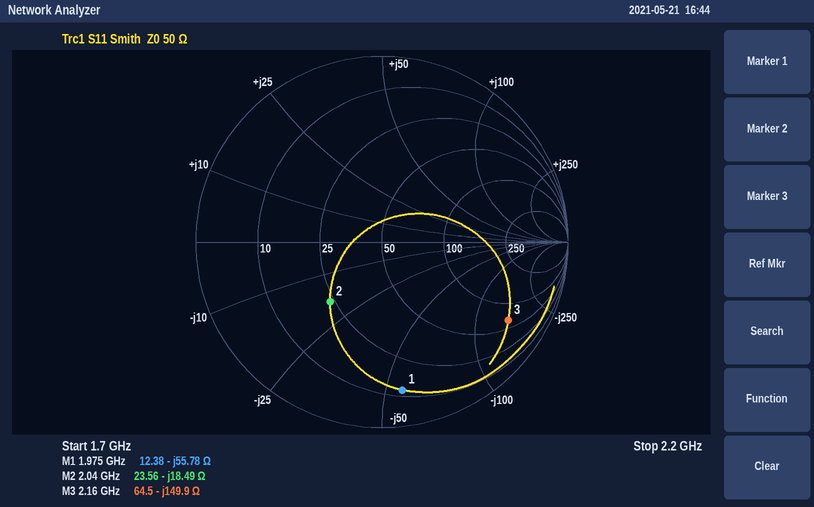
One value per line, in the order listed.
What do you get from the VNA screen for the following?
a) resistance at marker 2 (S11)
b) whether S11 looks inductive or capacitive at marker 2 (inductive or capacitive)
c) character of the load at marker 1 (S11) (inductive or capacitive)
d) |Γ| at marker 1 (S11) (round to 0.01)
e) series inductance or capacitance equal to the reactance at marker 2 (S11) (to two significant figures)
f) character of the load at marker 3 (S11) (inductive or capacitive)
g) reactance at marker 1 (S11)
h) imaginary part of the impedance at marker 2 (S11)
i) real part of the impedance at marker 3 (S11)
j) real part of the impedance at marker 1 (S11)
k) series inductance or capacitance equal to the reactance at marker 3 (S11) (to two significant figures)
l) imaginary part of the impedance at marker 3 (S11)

23.56 Ω
capacitive
capacitive
0.80
4.2 pF
capacitive
-55.78 Ω
-18.49 Ω
64.5 Ω
12.38 Ω
490 fF
-149.9 Ω
